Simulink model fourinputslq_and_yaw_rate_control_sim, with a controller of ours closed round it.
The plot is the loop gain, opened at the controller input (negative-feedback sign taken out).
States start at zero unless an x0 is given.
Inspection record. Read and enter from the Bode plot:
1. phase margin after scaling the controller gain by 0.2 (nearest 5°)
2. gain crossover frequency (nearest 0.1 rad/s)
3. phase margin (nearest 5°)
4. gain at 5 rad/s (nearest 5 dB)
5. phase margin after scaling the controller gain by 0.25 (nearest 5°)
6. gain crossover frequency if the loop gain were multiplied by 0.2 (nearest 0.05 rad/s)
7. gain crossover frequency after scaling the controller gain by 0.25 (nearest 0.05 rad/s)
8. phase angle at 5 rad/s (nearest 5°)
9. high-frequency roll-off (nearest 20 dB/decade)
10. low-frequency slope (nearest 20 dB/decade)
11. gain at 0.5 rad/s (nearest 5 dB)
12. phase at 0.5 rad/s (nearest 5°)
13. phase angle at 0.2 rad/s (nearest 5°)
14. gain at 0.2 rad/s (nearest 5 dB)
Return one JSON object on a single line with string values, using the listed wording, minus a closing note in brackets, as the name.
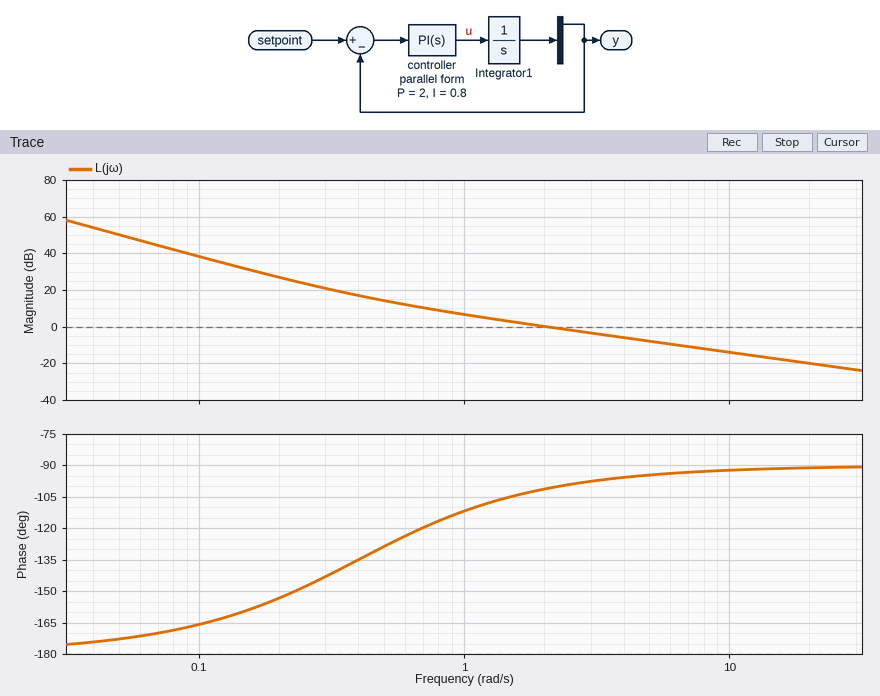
{"phase margin after scaling the controller gain by 0.2": "50°", "gain crossover frequency": "2.0 rad/s", "phase margin": "80°", "gain at 5 rad/s": "-10 dB", "phase margin after scaling the controller gain by 0.25": "55°", "gain crossover frequency if the loop gain were multiplied by 0.2": "0.50 rad/s", "gain crossover frequency after scaling the controller gain by 0.25": "0.60 rad/s", "phase angle at 5 rad/s": "-95°", "high-frequency roll-off": "-20 dB/decade", "low-frequency slope": "-40 dB/decade", "gain at 0.5 rad/s": "15 dB", "phase at 0.5 rad/s": "-130°", "phase angle at 0.2 rad/s": "-155°", "gain at 0.2 rad/s": "25 dB"}
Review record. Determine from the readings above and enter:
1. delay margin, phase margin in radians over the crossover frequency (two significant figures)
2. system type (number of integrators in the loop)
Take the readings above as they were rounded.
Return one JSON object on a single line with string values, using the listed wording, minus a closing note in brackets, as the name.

{"delay margin, phase margin in radians over the crossover frequency": "0.70 s", "system type": "2"}
